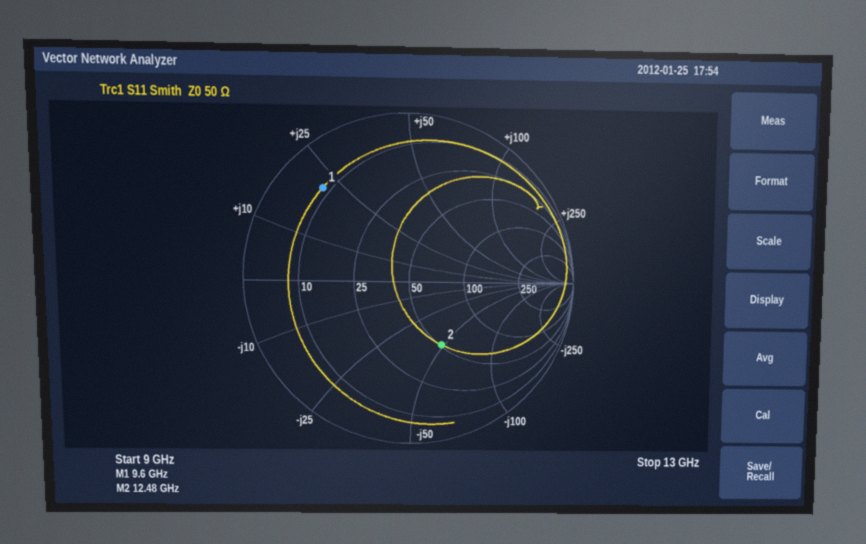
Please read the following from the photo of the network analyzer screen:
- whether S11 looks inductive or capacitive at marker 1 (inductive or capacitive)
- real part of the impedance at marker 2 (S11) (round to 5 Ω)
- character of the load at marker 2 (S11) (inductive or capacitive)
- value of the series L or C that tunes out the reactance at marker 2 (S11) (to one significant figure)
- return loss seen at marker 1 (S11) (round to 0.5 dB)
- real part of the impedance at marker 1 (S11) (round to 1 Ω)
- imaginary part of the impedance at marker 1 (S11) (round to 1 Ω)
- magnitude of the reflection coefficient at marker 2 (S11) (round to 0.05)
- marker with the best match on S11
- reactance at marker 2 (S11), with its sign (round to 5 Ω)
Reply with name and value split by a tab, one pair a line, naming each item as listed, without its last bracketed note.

whether S11 looks inductive or capacitive at marker 1	inductive
real part of the impedance at marker 2 (S11)	50 Ω
character of the load at marker 2 (S11)	capacitive
value of the series L or C that tunes out the reactance at marker 2 (S11)	600 pH
return loss seen at marker 1 (S11)	2.5 dB
real part of the impedance at marker 1 (S11)	8 Ω
imaginary part of the impedance at marker 1 (S11)	+21 Ω
magnitude of the reflection coefficient at marker 2 (S11)	0.45
marker with the best match on S11	marker 2
reactance at marker 2 (S11), with its sign	-50 Ω
